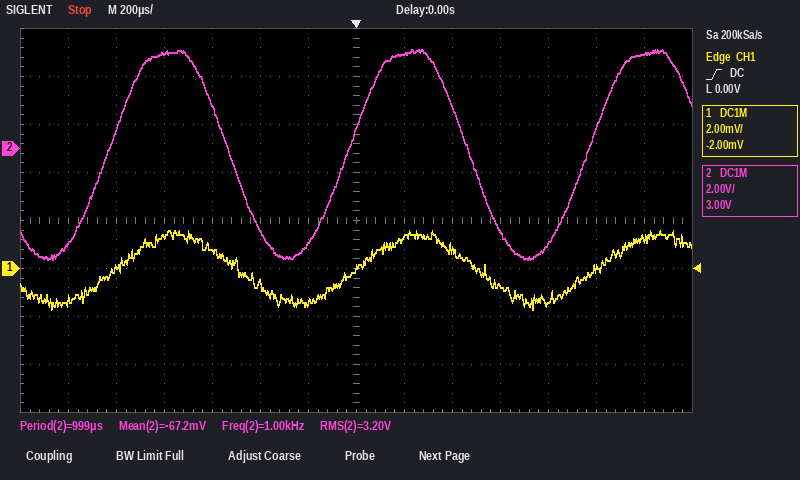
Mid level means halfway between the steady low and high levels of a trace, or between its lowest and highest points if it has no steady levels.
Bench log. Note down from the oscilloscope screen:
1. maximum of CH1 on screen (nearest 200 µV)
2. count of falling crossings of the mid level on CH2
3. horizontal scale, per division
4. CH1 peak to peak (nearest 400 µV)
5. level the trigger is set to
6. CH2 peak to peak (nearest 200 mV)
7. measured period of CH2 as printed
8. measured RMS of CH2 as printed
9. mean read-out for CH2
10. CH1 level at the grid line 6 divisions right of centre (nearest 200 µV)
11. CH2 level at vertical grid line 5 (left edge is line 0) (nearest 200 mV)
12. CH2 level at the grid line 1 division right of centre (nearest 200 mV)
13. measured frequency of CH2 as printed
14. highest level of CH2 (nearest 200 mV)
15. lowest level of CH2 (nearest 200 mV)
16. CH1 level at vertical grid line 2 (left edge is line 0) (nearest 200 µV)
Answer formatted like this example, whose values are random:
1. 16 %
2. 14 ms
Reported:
1. 1.6 mV
2. 2
3. 200 µs
4. 3.2 mV
5. 0.00 V
6. 8.8 V
7. 999 µs
8. 3.20 V
9. -67.2 mV
10. 1.2 mV
11. -3.4 V
12. 4.0 V
13. 1.00 kHz
14. 4.2 V
15. -4.6 V
16. 0.0 mV
